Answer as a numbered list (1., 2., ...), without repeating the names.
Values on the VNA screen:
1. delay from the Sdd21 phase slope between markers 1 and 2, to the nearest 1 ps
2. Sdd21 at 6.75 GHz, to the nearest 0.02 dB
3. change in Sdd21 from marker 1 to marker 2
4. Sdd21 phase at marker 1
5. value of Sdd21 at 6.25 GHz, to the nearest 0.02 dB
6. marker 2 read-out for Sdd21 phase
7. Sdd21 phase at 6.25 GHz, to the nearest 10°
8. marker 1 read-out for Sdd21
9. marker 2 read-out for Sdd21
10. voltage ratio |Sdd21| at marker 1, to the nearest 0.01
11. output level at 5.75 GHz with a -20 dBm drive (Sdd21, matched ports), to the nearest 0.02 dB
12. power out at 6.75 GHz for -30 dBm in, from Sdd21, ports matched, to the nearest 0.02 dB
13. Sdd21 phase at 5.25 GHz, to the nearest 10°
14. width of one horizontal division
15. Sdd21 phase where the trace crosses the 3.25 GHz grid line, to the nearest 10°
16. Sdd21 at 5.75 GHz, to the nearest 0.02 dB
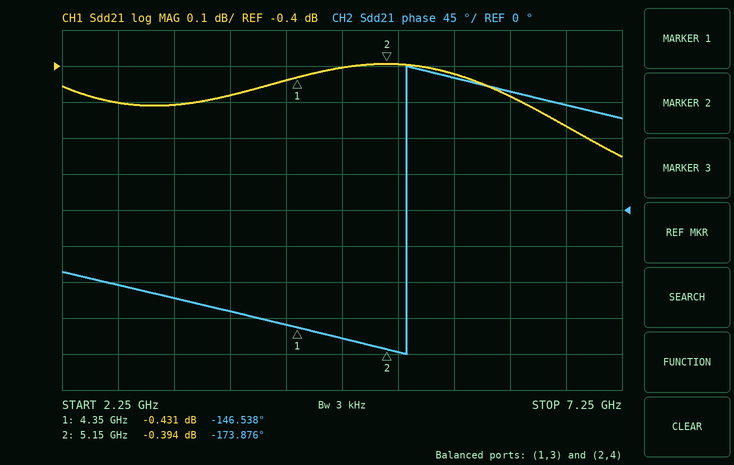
1. 95 ps
2. -0.56 dB
3. 0.037 dB
4. -146.538°
5. -0.48 dB
6. -173.876°
7. 150°
8. -0.431 dB
9. -0.394 dB
10. 0.95
11. -20.42 dBm
12. -30.56 dBm
13. -180°
14. 500 MHz
15. -110°
16. -0.42 dB
